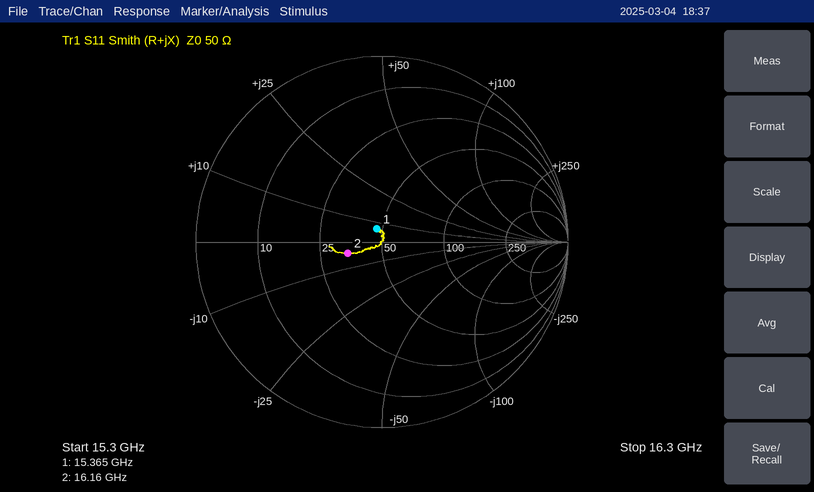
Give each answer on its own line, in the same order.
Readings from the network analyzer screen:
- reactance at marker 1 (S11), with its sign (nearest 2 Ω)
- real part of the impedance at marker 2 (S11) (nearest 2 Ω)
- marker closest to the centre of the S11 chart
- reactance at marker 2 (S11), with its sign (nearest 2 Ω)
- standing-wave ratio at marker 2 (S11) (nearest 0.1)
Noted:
+6 Ω
34 Ω
marker 1
-4 Ω
1.5
